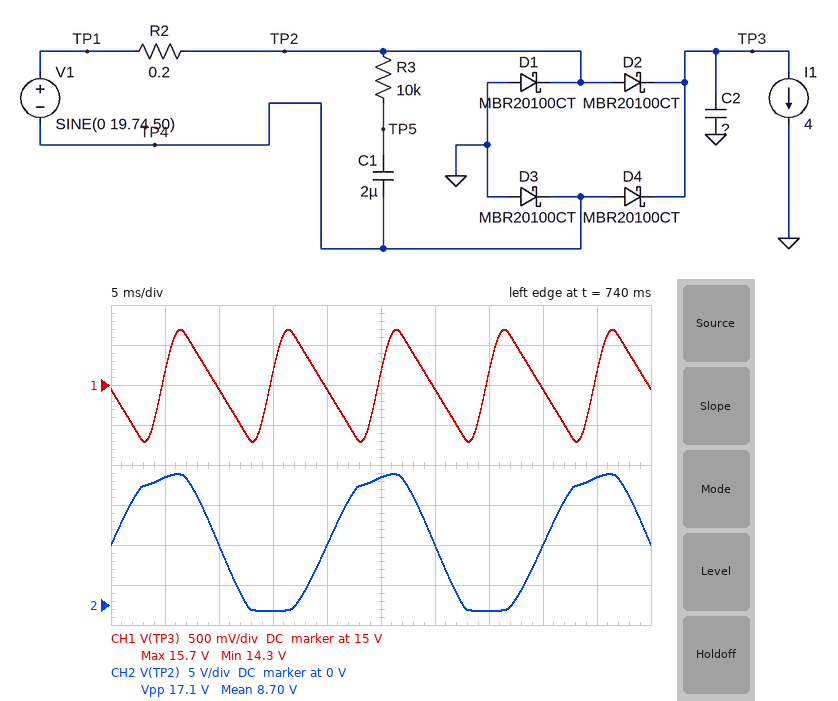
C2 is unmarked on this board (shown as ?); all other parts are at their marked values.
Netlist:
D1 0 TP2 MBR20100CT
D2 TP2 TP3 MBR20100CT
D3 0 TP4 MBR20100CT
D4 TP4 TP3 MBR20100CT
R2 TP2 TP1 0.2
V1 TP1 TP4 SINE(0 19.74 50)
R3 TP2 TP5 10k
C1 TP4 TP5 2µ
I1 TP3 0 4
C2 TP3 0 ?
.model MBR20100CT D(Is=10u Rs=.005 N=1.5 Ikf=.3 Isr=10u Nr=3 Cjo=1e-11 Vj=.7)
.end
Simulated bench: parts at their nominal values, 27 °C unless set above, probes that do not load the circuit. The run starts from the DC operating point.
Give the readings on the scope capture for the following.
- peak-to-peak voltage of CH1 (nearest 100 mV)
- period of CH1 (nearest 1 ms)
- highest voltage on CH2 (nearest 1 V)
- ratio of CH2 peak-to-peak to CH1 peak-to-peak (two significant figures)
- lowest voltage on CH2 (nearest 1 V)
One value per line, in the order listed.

1.4 V
10 ms
16 V
12
-1 V
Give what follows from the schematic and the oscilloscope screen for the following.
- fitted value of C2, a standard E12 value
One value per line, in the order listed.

18 mF
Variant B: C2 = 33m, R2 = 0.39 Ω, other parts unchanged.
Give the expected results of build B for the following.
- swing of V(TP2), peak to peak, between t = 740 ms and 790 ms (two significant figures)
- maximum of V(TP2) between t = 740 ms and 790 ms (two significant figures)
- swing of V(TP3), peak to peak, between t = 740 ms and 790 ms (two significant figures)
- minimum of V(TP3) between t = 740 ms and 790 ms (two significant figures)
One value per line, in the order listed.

15 V
14 V
680 mV
13 V
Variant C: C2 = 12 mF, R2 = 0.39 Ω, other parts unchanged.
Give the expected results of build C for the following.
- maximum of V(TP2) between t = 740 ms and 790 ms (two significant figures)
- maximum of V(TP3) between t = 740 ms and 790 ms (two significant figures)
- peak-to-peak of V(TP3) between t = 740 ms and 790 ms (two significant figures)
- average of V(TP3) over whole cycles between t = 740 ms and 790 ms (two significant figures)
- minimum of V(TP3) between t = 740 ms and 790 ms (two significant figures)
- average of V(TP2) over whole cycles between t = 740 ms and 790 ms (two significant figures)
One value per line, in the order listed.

15 V
14 V
1.9 V
13 V
12 V
6.6 V
